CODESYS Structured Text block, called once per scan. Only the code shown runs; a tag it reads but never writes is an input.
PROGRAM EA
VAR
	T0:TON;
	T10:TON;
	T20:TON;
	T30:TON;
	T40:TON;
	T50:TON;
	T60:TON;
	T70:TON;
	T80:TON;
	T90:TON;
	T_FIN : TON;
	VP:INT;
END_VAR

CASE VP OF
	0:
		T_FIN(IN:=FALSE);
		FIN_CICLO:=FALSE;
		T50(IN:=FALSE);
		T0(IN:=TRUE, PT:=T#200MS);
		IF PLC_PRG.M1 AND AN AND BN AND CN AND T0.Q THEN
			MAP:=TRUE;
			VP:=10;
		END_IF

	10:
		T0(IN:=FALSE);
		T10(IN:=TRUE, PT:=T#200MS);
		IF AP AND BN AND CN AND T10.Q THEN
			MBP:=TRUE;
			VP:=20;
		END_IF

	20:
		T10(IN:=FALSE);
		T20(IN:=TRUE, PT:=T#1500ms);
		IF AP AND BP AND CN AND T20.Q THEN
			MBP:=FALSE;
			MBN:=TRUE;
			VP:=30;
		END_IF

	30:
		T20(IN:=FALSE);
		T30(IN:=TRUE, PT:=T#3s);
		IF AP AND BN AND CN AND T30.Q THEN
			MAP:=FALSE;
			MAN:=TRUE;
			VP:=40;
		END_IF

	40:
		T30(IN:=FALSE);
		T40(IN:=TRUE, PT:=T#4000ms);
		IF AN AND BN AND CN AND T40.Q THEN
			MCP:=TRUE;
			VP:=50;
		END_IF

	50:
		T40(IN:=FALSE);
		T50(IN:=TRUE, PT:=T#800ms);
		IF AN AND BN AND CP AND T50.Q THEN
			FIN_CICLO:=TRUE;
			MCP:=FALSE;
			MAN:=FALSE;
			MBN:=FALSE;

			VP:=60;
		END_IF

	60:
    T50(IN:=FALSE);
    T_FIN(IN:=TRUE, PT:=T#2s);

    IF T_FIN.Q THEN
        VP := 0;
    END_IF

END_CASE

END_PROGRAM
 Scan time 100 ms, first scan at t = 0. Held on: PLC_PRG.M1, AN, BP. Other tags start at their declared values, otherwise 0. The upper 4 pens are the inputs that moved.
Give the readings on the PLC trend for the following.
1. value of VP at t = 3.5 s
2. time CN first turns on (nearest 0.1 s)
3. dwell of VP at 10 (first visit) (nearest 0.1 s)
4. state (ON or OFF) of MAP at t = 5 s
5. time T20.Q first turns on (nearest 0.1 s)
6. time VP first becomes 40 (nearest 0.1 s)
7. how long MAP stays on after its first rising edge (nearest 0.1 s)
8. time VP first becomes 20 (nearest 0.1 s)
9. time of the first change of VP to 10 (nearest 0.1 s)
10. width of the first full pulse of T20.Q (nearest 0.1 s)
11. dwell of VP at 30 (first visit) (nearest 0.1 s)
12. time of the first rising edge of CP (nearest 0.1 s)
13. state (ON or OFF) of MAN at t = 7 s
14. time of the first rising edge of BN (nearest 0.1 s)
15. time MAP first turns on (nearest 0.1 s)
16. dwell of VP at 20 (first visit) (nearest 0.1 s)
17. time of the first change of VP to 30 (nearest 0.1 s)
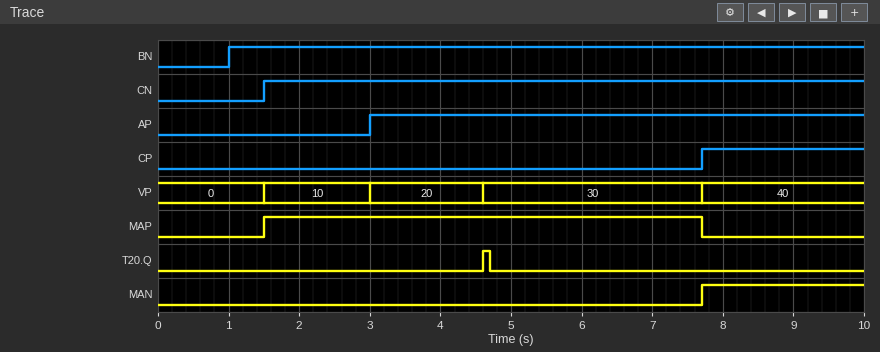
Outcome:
20
1.5 s
1.5 s
ON
4.6 s
7.7 s
6.2 s
3.0 s
1.5 s
0.1 s
3.1 s
7.7 s
OFF
1.0 s
1.5 s
1.6 s
4.6 s
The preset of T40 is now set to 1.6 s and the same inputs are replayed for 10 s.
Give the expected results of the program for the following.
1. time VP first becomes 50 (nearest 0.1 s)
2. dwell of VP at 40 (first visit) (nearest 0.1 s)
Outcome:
9.4 s
1.7 s
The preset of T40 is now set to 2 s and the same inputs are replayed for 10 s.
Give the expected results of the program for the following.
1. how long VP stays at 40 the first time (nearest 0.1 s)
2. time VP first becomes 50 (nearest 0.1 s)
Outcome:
2.1 s
9.8 s
